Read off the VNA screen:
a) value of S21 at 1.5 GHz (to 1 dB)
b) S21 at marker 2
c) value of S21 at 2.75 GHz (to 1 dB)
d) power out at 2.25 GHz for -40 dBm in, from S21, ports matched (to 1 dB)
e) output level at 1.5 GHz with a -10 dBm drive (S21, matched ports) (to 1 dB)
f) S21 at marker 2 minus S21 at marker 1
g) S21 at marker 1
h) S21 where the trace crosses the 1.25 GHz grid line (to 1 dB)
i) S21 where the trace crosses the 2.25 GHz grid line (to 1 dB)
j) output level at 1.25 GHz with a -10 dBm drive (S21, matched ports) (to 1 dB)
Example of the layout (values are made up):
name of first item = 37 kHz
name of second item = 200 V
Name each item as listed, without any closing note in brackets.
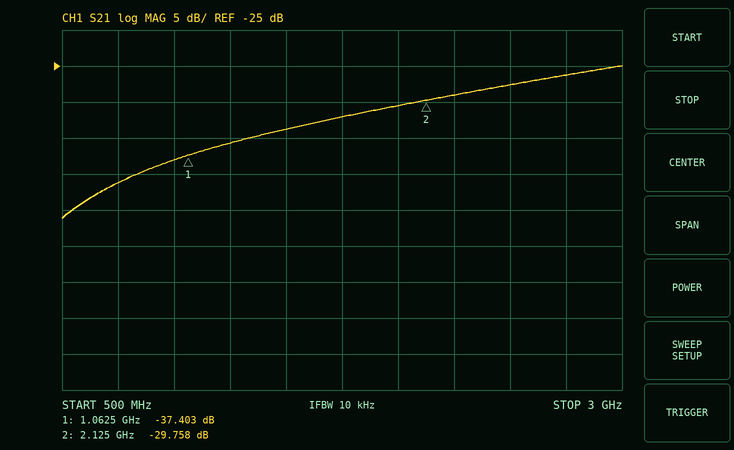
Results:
value of S21 at 1.5 GHz = -34 dB
S21 at marker 2 = -29.758 dB
value of S21 at 2.75 GHz = -26 dB
power out at 2.25 GHz for -40 dBm in, from S21, ports matched = -69 dBm
output level at 1.5 GHz with a -10 dBm drive (S21, matched ports) = -44 dBm
S21 at marker 2 minus S21 at marker 1 = 7.645 dB
S21 at marker 1 = -37.403 dB
S21 where the trace crosses the 1.25 GHz grid line = -36 dB
S21 where the trace crosses the 2.25 GHz grid line = -29 dB
output level at 1.25 GHz with a -10 dBm drive (S21, matched ports) = -46 dBm
